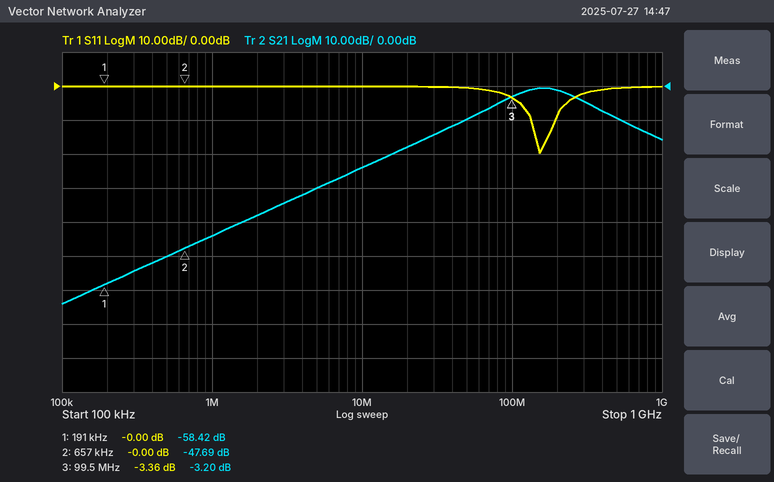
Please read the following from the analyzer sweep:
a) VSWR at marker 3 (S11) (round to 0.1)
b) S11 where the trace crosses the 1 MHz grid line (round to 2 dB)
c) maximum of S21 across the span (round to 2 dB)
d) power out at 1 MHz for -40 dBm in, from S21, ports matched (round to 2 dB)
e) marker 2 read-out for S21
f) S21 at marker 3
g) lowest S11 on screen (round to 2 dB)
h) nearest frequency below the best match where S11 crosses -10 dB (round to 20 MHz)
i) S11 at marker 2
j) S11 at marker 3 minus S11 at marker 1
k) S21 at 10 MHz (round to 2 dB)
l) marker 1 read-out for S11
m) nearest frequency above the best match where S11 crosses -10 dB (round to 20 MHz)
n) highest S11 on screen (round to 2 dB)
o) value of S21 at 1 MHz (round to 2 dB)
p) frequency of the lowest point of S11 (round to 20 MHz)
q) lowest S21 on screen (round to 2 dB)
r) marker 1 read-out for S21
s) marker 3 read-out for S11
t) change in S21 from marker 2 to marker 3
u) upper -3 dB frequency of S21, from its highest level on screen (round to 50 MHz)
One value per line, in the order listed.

5.2
0 dB
0 dB
-84 dBm
-47.69 dB
-3.20 dB
-20 dB
140 MHz
-0.00 dB
-3.36 dB
-24 dB
-0.00 dB
200 MHz
0 dB
-44 dB
160 MHz
-64 dB
-58.42 dB
-3.36 dB
44.49 dB
250 MHz
